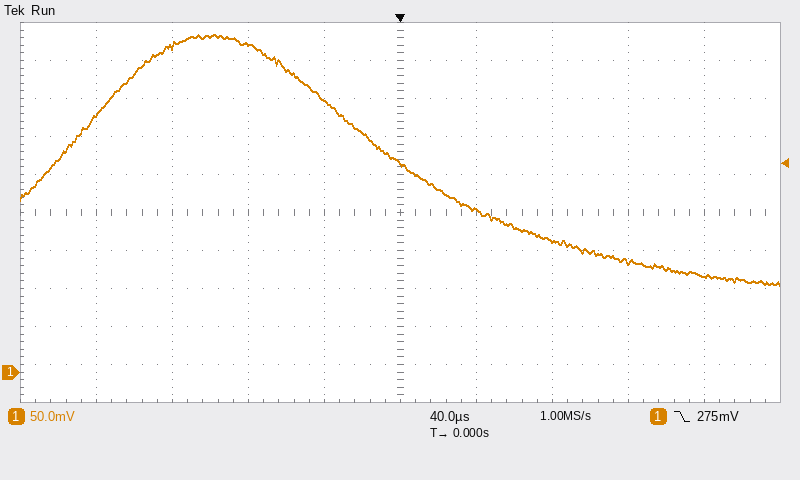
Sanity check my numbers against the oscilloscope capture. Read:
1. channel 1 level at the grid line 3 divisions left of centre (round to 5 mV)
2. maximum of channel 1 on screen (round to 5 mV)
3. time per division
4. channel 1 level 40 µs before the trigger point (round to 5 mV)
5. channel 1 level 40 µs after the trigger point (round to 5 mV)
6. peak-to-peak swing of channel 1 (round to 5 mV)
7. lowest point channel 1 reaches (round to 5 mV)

430 mV
445 mV
40 µs
355 mV
215 mV
330 mV
115 mV
